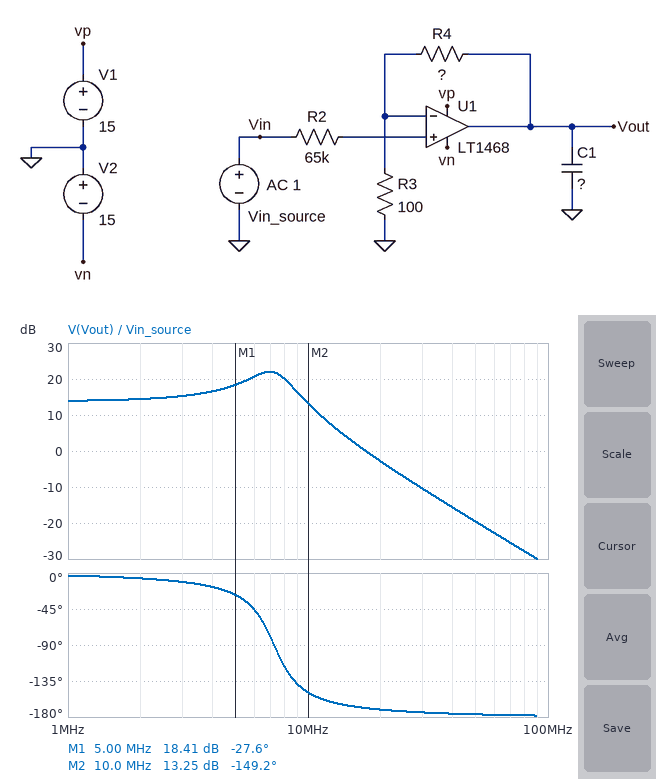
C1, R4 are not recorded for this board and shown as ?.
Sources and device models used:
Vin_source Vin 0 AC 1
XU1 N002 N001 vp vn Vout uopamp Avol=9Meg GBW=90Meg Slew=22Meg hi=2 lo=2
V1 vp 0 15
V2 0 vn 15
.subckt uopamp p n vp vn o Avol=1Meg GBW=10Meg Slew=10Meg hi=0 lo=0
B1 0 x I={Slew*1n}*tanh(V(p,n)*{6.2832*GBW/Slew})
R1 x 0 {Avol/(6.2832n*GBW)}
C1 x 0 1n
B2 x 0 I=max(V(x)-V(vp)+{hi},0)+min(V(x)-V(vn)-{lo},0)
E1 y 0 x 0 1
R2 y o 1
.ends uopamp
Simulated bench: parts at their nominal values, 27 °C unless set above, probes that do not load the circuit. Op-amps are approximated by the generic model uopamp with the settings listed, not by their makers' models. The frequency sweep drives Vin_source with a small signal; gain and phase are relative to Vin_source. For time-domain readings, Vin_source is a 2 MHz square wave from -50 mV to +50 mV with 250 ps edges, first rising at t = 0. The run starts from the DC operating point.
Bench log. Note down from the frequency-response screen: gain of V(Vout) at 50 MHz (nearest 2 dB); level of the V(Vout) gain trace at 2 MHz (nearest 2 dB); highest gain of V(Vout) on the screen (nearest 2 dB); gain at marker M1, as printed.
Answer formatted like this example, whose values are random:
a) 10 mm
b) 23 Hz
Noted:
a) -20 dB
b) 14 dB
c) 22 dB
d) 18.41 dB
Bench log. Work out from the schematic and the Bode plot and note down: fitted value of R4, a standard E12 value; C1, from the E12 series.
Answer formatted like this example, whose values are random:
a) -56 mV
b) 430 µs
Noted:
a) 390 Ω
b) 56 nF
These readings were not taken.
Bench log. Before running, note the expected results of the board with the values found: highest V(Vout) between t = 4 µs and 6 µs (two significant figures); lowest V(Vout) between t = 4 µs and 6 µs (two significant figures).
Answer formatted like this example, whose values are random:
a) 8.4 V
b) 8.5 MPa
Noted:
a) 450 mV
b) -450 mV
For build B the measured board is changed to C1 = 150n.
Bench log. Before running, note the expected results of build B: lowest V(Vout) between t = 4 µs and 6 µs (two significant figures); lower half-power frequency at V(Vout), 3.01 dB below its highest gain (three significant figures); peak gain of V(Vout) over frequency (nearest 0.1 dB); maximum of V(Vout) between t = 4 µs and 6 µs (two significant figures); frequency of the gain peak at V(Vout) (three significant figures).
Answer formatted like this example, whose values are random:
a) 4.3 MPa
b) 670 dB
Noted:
a) -460 mV
b) 3.78 MHz
c) 26.2 dB
d) 460 mV
e) 4.35 MHz
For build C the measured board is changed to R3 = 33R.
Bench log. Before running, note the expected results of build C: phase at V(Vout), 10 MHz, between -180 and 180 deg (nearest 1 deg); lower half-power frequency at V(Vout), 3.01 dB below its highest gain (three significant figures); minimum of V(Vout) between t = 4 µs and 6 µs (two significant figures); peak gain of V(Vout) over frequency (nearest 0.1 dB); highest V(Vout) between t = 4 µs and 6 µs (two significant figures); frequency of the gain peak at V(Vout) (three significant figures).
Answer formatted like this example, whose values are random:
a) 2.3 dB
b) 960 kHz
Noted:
a) -160 deg
b) 1.96 MHz
c) -920 mV
d) 26.5 dB
e) 920 mV
f) 3.99 MHz
